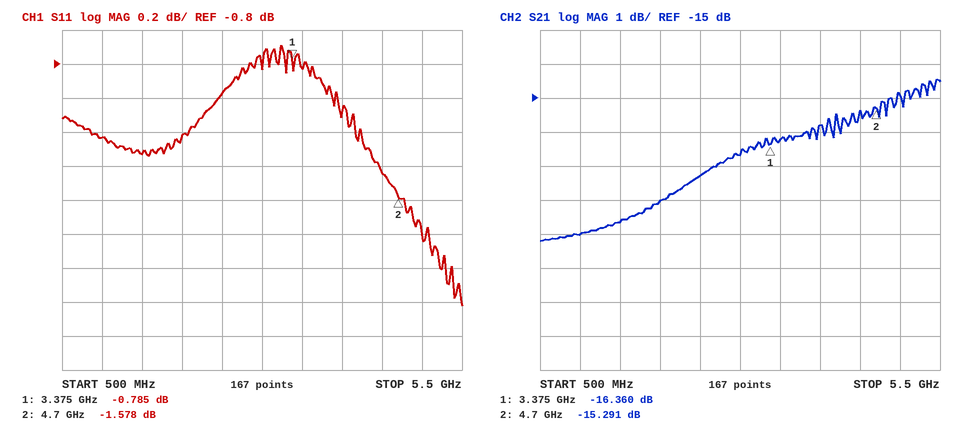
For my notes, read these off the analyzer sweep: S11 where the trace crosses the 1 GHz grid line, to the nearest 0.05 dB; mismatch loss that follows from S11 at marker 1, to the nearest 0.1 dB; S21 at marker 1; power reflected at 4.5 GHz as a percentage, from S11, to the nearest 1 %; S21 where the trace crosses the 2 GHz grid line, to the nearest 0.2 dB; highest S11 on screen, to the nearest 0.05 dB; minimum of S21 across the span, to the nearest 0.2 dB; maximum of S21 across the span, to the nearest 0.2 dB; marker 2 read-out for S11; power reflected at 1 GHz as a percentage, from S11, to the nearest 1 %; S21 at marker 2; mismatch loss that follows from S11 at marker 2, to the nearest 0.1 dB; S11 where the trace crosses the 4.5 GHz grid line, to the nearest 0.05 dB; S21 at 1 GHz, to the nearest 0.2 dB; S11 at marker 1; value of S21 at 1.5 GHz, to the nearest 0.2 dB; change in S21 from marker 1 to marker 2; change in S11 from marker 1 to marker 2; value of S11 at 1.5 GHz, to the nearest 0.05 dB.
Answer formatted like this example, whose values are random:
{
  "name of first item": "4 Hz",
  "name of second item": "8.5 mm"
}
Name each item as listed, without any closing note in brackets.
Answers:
{
  "S11 where the trace crosses the 1 GHz grid line, to the nearest 0.05 dB": "-1.25 dB",
  "mismatch loss that follows from S11 at marker 1, to the nearest 0.1 dB": "7.8 dB",
  "S21 at marker 1": "-16.360 dB",
  "power reflected at 4.5 GHz as a percentage, from S11, to the nearest 1 %": "72 %",
  "S21 where the trace crosses the 2 GHz grid line, to the nearest 0.2 dB": "-18.0 dB",
  "highest S11 on screen, to the nearest 0.05 dB": "-0.70 dB",
  "minimum of S21 across the span, to the nearest 0.2 dB": "-19.2 dB",
  "maximum of S21 across the span, to the nearest 0.2 dB": "-14.4 dB",
  "marker 2 read-out for S11": "-1.578 dB",
  "power reflected at 1 GHz as a percentage, from S11, to the nearest 1 %": "75 %",
  "S21 at marker 2": "-15.291 dB",
  "mismatch loss that follows from S11 at marker 2, to the nearest 0.1 dB": "5.2 dB",
  "S11 where the trace crosses the 4.5 GHz grid line, to the nearest 0.05 dB": "-1.45 dB",
  "S21 at 1 GHz, to the nearest 0.2 dB": "-19.0 dB",
  "S11 at marker 1": "-0.785 dB",
  "value of S21 at 1.5 GHz, to the nearest 0.2 dB": "-18.6 dB",
  "change in S21 from marker 1 to marker 2": "1.069 dB",
  "change in S11 from marker 1 to marker 2": "-0.793 dB",
  "value of S11 at 1.5 GHz, to the nearest 0.05 dB": "-1.35 dB"
}
